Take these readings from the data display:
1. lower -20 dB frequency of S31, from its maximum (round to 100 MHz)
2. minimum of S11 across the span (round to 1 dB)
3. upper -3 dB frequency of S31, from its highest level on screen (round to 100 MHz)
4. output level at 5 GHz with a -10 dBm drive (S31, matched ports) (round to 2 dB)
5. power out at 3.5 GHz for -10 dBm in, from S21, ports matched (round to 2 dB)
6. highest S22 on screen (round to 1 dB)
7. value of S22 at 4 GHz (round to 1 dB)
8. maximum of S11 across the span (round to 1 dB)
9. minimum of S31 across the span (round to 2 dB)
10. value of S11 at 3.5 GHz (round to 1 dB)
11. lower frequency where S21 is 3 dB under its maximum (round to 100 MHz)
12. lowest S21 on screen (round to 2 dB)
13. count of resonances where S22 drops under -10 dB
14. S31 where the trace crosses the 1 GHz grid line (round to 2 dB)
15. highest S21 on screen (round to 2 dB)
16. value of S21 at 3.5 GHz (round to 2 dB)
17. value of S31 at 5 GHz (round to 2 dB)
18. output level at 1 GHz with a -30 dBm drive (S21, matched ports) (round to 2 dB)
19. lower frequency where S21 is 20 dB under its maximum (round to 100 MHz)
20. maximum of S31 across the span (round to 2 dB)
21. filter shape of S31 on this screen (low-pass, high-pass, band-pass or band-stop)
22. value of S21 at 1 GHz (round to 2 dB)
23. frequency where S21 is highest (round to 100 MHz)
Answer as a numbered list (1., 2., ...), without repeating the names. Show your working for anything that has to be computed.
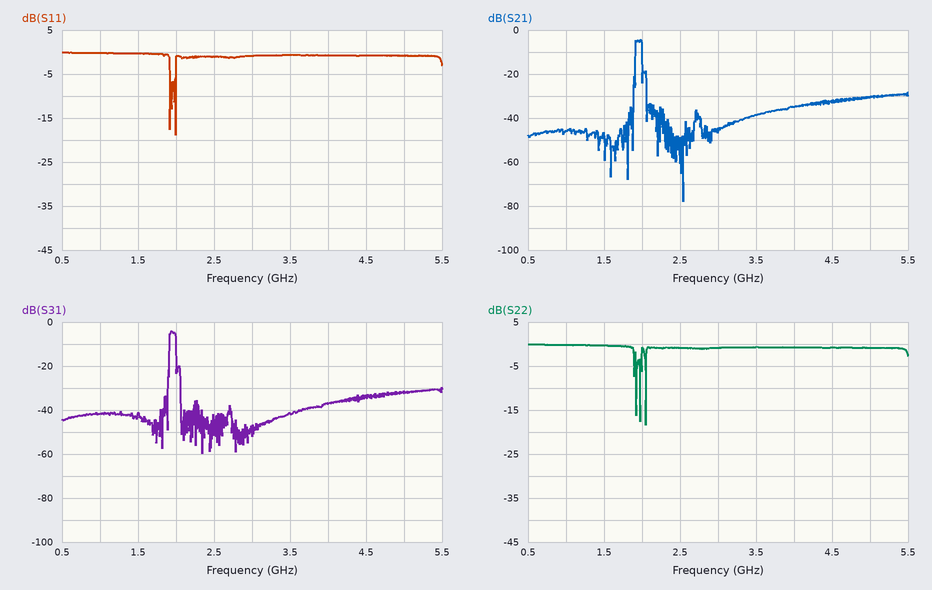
1. 1.9 GHz
2. -19 dB
3. 2.0 GHz
4. -10 dBm + (-32 dB) = -42 dBm
5. -10 dBm + (-38 dB) = -48 dBm
6. 0 dB
7. -1 dB
8. 0 dB
9. -60 dB
10. -1 dB
11. 1.9 GHz
12. -78 dB
13. 3
14. -42 dB
15. -4 dB
16. -38 dB
17. -32 dB
18. -30 dBm + (-46 dB) = -76 dBm
19. 1.9 GHz
20. -4 dB
21. band-pass
22. -46 dB
23. 2.0 GHz
